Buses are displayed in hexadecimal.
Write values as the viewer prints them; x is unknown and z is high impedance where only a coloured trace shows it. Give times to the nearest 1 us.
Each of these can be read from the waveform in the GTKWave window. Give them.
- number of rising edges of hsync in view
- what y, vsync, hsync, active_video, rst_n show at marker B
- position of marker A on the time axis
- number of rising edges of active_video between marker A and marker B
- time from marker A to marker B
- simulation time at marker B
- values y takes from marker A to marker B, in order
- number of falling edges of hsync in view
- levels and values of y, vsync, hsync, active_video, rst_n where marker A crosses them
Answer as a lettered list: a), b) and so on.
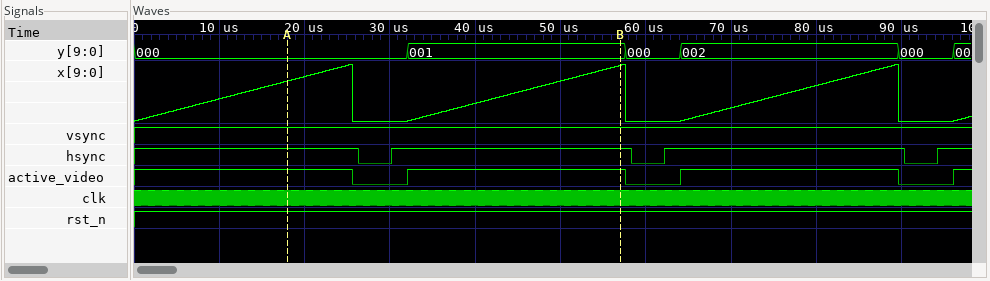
a) 3
b) y=001, vsync=1, hsync=1, active_video=1, rst_n=1
c) 18 us
d) 1
e) 39 us
f) 57 us
g) 000, 001
h) 3
i) y=000, vsync=1, hsync=1, active_video=1, rst_n=1
